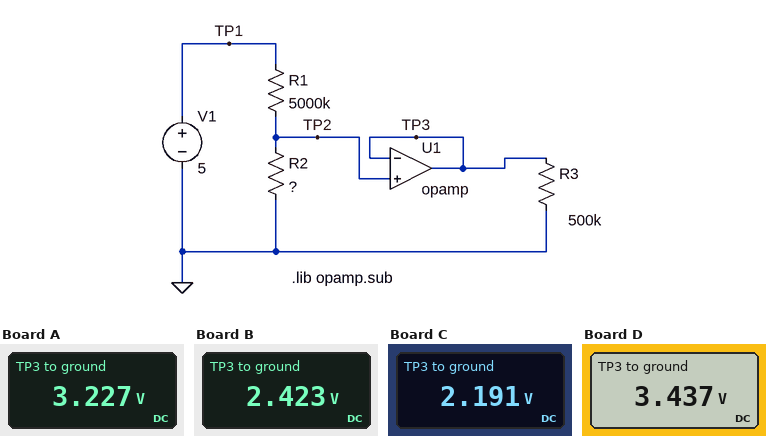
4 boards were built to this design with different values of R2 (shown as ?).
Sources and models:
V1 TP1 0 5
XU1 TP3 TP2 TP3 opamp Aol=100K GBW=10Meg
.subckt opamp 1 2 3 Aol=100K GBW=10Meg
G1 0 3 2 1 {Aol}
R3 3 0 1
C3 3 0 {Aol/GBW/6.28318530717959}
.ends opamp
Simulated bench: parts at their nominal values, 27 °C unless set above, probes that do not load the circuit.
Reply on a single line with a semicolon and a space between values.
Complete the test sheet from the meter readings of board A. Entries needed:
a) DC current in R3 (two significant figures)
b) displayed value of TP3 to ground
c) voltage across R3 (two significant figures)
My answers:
6.5 µA; 3.227 V; 3.2 V
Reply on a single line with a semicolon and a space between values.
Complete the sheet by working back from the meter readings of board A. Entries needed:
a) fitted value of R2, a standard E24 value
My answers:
9.1 MΩ
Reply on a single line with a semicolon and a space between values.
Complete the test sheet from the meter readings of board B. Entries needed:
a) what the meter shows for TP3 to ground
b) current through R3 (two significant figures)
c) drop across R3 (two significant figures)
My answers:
2.423 V; 4.8 µA; 2.4 V
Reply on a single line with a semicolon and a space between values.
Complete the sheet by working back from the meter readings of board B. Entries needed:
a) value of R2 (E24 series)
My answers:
4.7 MΩ
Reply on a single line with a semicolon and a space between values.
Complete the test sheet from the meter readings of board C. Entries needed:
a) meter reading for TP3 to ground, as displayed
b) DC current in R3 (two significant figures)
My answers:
2.191 V; 4.4 µA
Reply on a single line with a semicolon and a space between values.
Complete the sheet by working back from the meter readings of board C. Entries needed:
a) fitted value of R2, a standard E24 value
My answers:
3.9 MΩ
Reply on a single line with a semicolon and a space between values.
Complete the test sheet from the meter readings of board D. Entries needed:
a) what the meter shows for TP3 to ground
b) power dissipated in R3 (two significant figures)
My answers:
3.437 V; 24 µW
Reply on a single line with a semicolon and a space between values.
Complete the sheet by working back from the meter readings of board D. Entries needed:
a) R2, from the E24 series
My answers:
11 MΩ
